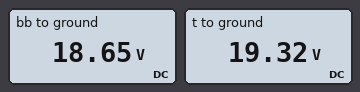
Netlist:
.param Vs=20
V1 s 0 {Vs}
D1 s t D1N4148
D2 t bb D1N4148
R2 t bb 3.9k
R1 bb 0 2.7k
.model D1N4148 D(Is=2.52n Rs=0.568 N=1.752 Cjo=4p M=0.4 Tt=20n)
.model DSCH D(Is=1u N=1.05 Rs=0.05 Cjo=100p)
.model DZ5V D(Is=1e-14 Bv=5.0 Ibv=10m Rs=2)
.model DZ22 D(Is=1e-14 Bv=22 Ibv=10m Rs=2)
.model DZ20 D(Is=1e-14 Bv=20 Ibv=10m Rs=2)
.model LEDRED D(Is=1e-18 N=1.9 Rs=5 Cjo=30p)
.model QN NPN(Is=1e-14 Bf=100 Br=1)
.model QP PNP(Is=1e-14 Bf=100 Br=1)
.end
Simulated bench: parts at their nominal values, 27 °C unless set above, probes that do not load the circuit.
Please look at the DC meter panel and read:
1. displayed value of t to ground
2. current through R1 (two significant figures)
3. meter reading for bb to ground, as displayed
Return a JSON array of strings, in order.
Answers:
["19.32 V", "6.9 mA", "18.65 V"]
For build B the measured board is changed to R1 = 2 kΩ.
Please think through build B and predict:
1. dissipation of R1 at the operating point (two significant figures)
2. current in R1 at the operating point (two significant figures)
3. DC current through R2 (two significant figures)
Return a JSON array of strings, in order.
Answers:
["170 mW", "9.3 mA", "180 µA"]
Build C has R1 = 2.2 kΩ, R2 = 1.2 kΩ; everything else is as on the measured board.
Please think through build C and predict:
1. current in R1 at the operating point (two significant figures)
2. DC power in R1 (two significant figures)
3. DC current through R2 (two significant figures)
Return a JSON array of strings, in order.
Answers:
["8.5 mA", "160 mW", "570 µA"]
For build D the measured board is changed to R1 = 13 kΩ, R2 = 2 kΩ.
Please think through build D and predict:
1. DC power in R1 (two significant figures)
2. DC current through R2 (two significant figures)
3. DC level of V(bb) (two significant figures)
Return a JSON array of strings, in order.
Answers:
["27 mW", "300 µA", "19 V"]
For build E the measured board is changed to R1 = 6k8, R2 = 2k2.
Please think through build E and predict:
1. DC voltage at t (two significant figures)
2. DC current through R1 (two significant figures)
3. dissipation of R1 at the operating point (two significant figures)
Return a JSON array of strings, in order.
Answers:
["19 V", "2.8 mA", "52 mW"]
